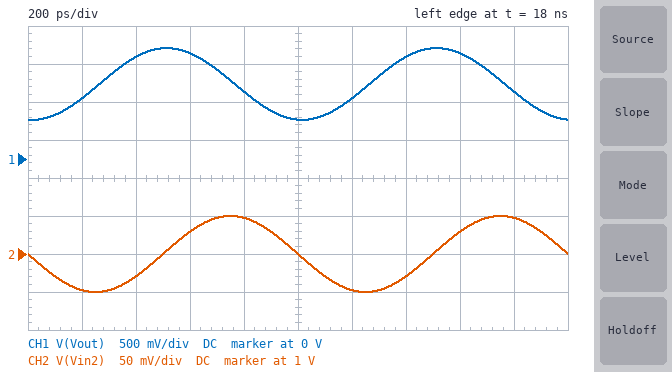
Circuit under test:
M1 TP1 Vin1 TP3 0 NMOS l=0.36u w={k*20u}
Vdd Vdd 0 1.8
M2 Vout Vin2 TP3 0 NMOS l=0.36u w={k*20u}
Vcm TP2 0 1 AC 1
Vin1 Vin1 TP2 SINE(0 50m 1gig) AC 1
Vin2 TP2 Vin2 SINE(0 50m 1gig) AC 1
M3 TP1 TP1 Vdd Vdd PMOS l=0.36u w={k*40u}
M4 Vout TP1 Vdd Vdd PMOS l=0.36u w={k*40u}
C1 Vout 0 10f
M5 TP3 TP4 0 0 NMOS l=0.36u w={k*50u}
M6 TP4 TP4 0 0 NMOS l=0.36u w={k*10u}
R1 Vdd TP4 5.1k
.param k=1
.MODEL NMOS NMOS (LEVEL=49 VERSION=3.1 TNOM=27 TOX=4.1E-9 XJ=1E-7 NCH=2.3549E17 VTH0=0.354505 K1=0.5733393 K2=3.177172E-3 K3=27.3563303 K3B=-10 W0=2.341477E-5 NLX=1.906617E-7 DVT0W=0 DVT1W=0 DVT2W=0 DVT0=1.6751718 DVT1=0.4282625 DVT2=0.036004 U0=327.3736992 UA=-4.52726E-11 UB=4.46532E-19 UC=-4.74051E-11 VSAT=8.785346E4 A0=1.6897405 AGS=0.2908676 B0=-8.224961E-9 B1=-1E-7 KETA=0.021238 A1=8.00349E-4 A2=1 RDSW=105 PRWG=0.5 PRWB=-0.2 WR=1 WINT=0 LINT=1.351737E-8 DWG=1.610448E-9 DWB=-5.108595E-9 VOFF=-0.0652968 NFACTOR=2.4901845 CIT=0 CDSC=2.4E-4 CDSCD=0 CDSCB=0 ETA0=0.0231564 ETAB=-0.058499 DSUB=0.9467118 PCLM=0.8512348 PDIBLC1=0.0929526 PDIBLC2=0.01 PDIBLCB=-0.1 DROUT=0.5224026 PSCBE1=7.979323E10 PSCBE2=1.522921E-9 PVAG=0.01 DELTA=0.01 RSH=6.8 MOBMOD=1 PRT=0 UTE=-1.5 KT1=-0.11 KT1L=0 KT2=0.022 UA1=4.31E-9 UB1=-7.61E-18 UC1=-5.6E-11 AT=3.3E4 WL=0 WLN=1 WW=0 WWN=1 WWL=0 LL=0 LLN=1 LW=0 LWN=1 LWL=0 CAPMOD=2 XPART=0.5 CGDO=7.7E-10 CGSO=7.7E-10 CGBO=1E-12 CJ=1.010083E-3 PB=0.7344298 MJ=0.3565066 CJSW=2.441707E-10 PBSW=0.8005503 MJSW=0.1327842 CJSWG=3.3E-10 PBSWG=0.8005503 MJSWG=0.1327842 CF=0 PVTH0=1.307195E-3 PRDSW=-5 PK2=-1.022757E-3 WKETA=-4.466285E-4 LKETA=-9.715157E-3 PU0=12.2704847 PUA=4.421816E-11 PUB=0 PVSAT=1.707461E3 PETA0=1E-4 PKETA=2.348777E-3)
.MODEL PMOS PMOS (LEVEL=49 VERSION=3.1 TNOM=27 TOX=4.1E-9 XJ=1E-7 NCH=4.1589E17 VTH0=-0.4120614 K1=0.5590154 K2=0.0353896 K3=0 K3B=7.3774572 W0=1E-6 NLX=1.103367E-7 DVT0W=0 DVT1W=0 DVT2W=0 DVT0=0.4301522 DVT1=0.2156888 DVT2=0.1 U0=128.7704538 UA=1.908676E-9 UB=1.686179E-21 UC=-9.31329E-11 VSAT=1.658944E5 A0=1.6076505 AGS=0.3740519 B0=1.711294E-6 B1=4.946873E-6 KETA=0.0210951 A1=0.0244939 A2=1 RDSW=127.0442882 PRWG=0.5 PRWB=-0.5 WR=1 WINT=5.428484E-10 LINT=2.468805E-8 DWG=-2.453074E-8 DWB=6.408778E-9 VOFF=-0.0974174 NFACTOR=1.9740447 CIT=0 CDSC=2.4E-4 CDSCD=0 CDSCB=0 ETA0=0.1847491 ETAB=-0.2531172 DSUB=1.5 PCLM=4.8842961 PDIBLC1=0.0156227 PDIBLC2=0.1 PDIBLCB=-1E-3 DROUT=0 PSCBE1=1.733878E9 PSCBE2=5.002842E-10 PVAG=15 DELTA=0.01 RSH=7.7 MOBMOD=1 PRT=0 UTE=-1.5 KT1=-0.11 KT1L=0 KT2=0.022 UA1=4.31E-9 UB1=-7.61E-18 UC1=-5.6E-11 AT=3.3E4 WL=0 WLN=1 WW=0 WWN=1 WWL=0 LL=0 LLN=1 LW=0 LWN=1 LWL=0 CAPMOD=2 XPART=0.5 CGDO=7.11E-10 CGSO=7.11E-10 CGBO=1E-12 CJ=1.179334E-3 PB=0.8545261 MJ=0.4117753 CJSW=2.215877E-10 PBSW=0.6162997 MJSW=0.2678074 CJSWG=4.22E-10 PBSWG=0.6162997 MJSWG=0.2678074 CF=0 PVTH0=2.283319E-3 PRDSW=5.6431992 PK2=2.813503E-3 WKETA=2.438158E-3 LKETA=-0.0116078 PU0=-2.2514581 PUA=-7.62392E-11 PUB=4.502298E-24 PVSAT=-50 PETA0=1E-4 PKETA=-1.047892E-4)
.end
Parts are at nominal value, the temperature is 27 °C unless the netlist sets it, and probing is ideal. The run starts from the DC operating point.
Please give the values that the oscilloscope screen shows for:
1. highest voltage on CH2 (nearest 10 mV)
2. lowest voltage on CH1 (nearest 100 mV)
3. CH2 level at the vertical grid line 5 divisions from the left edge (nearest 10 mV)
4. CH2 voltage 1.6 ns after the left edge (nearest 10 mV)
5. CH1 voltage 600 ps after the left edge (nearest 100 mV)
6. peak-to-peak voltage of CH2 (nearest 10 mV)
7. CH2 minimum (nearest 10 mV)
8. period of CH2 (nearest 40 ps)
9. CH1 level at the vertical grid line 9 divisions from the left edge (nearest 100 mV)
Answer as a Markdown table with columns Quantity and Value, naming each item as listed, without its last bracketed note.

| Quantity | Value |
|---|---|
| highest voltage on CH2 | 1.05 V |
| lowest voltage on CH1 | 500 mV |
| CH2 level at the vertical grid line 5 divisions from the left edge | 1.00 V |
| CH2 voltage 1.6 ns after the left edge | 1.03 V |
| CH1 voltage 600 ps after the left edge | 1.4 V |
| peak-to-peak voltage of CH2 | 100 mV |
| CH2 minimum | 950 mV |
| period of CH2 | 1.00 ns |
| CH1 level at the vertical grid line 9 divisions from the left edge | 900 mV |
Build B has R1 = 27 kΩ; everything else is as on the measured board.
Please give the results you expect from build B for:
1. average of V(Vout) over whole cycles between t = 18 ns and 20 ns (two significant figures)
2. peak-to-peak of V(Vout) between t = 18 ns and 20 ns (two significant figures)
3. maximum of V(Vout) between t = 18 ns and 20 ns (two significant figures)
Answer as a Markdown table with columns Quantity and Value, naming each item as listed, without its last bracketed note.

| Quantity | Value |
|---|---|
| average of V(Vout) over whole cycles between t = 18 ns and 20 ns | 1.2 V |
| peak-to-peak of V(Vout) between t = 18 ns and 20 ns | 400 mV |
| maximum of V(Vout) between t = 18 ns and 20 ns | 1.4 V |
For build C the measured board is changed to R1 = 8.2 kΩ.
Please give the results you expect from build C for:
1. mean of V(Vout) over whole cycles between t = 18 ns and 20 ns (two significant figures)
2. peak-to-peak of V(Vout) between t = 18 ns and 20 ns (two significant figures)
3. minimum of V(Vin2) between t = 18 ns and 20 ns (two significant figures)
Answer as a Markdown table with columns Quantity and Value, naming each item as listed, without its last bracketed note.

| Quantity | Value |
|---|---|
| mean of V(Vout) over whole cycles between t = 18 ns and 20 ns | 1.0 V |
| peak-to-peak of V(Vout) between t = 18 ns and 20 ns | 810 mV |
| minimum of V(Vin2) between t = 18 ns and 20 ns | 950 mV |
